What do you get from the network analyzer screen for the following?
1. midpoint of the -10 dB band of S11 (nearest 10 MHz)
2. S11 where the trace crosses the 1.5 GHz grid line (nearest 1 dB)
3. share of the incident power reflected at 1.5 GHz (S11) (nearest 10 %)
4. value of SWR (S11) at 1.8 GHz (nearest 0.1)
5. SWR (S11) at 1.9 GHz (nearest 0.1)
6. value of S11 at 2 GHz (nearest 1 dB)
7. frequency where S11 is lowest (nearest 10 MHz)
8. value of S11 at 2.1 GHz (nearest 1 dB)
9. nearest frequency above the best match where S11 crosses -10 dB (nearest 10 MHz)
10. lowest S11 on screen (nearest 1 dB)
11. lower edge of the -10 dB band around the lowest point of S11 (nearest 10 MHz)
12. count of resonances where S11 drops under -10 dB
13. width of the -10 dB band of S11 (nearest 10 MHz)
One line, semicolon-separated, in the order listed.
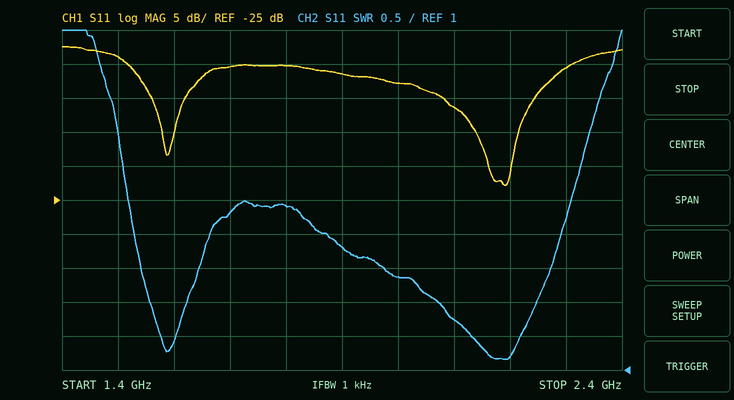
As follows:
2.16 GHz; -4 dB; 40 %; 3.4; 2.8; -8 dB; 2.19 GHz; -11 dB; 2.24 GHz; -23 dB; 2.08 GHz; 2; 160 MHz
